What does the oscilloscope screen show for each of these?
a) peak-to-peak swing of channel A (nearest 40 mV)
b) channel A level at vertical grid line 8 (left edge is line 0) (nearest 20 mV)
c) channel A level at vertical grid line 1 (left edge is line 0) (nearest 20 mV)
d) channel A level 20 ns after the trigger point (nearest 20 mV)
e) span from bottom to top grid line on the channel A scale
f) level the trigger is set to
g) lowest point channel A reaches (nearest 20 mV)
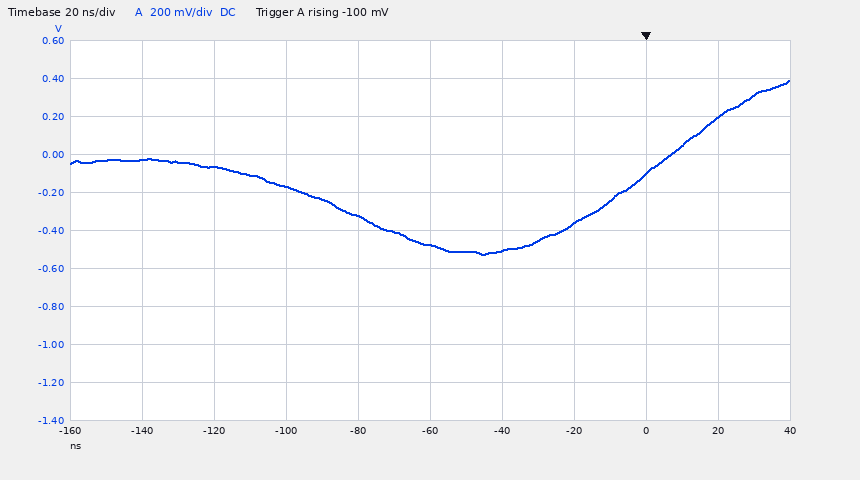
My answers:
920 mV
-100 mV
-20 mV
200 mV
2 V
-100 mV
-520 mV
